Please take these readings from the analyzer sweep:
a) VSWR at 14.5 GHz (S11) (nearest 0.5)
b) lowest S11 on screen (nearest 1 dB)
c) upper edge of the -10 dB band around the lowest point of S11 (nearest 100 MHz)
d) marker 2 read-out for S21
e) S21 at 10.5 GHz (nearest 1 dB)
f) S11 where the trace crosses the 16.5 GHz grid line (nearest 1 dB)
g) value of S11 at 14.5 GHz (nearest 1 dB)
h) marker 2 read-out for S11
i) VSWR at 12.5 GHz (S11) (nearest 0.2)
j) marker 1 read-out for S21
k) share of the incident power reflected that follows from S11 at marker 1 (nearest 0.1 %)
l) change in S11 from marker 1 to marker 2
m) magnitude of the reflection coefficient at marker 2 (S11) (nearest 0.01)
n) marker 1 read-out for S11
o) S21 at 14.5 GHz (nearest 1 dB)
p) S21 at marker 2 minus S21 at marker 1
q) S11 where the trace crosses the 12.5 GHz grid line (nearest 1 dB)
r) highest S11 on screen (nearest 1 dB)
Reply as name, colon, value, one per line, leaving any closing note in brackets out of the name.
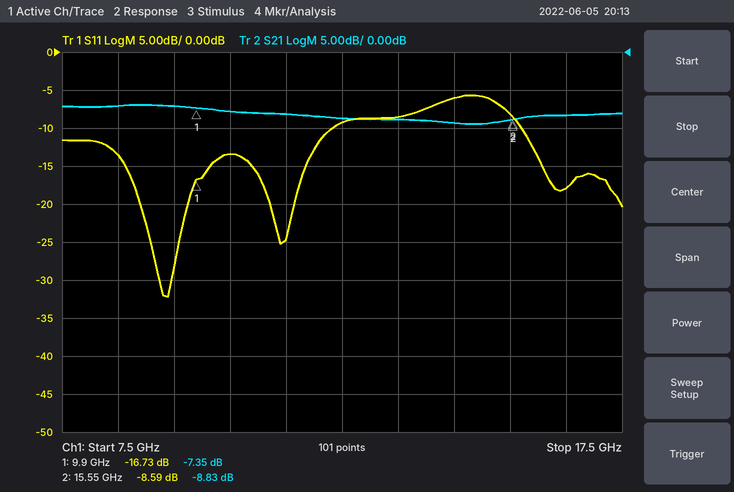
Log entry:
VSWR at 14.5 GHz (S11): 3.0
lowest S11 on screen: -32 dB
upper edge of the -10 dB band around the lowest point of S11: 12.3 GHz
marker 2 read-out for S21: -8.83 dB
S21 at 10.5 GHz: -8 dB
S11 where the trace crosses the 16.5 GHz grid line: -18 dB
value of S11 at 14.5 GHz: -6 dB
marker 2 read-out for S11: -8.59 dB
VSWR at 12.5 GHz (S11): 2.0
marker 1 read-out for S21: -7.35 dB
share of the incident power reflected that follows from S11 at marker 1: 2.1 %
change in S11 from marker 1 to marker 2: 8.14 dB
magnitude of the reflection coefficient at marker 2 (S11): 0.37
marker 1 read-out for S11: -16.73 dB
S21 at 14.5 GHz: -9 dB
S21 at marker 2 minus S21 at marker 1: -1.48 dB
S11 where the trace crosses the 12.5 GHz grid line: -9 dB
highest S11 on screen: -6 dB
